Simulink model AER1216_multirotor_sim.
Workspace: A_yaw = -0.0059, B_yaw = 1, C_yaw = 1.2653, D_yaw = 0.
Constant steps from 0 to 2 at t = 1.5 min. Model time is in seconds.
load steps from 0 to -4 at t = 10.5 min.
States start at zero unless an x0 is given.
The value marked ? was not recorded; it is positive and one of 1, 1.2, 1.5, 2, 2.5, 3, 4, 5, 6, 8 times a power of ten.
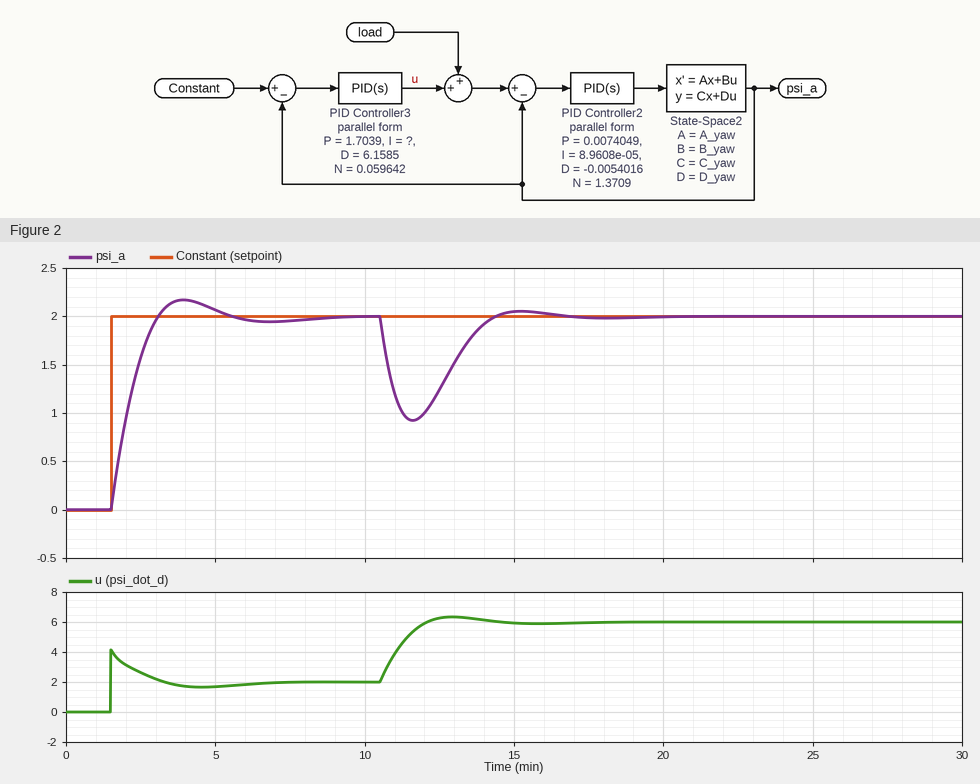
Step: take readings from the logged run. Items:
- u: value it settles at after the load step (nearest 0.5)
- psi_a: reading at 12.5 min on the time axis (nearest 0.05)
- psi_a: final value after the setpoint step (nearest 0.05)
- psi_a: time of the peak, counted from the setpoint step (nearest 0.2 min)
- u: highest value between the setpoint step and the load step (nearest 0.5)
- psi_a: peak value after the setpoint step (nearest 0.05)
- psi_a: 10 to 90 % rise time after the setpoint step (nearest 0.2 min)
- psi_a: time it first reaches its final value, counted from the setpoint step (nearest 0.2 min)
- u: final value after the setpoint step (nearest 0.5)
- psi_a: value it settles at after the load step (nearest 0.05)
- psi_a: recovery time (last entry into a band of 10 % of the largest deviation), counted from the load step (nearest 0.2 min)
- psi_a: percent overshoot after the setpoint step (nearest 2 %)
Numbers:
6.0
1.25
2.00
2.4 min
4.0
2.15
1.2 min
1.6 min
2.0
2.00
3.4 min
8 %
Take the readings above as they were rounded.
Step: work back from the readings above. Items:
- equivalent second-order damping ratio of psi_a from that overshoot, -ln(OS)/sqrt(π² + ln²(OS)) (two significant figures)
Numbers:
0.63
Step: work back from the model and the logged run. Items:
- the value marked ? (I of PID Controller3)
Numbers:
0.03
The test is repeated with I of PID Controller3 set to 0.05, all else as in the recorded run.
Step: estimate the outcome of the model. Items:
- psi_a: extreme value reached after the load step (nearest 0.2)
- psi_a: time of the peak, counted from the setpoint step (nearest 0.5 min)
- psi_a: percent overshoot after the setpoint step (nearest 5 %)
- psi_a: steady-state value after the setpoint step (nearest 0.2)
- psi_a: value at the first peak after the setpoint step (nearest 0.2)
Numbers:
1.0
2.0 min
20 %
2.0
2.4
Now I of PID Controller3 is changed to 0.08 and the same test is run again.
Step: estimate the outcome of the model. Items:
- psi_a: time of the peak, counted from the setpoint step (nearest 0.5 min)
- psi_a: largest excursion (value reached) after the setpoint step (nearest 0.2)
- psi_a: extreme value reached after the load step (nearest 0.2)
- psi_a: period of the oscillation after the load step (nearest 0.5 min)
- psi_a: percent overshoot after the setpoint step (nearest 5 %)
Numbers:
1.5 min
2.6
1.2
4.0 min
30 %
